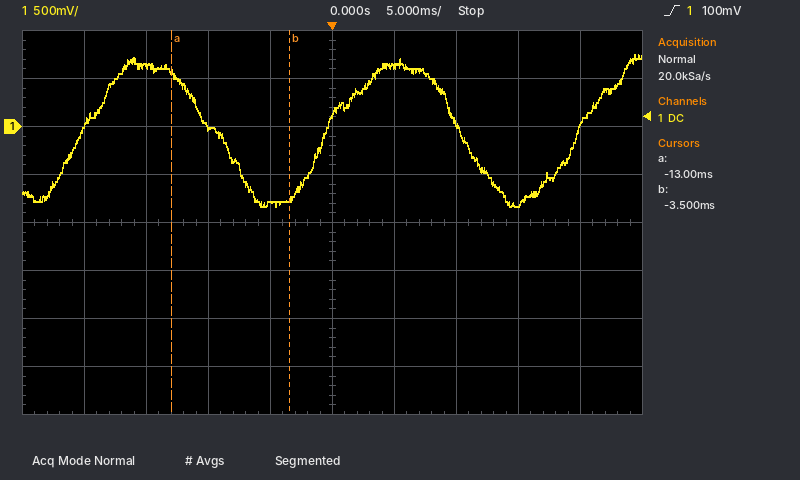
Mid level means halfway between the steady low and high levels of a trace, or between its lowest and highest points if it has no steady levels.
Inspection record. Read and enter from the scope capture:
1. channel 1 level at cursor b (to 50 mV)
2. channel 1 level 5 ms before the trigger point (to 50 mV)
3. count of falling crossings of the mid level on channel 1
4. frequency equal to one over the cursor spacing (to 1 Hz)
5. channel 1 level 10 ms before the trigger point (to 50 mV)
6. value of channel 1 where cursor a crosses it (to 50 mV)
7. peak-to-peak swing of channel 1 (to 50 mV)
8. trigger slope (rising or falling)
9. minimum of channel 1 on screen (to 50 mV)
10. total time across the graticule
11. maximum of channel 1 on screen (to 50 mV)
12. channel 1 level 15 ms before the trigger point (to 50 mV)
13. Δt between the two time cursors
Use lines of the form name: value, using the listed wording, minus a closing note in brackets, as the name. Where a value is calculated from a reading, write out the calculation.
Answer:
channel 1 level at cursor b: -750 mV
channel 1 level 5 ms before the trigger point: -800 mV
count of falling crossings of the mid level on channel 1: 2
frequency equal to one over the cursor spacing: 1 / 9.5 ms ≈ 105 Hz
channel 1 level 10 ms before the trigger point: 0 mV
value of channel 1 where cursor a crosses it: 550 mV
peak-to-peak swing of channel 1: 750 mV − (-850 mV) = 1.60 V
trigger slope: rising
minimum of channel 1 on screen: -850 mV
total time across the graticule: 50 ms
maximum of channel 1 on screen: 750 mV
channel 1 level 15 ms before the trigger point: 650 mV
Δt between the two time cursors: -3.5 ms − (-13 ms) = 9.5 ms
